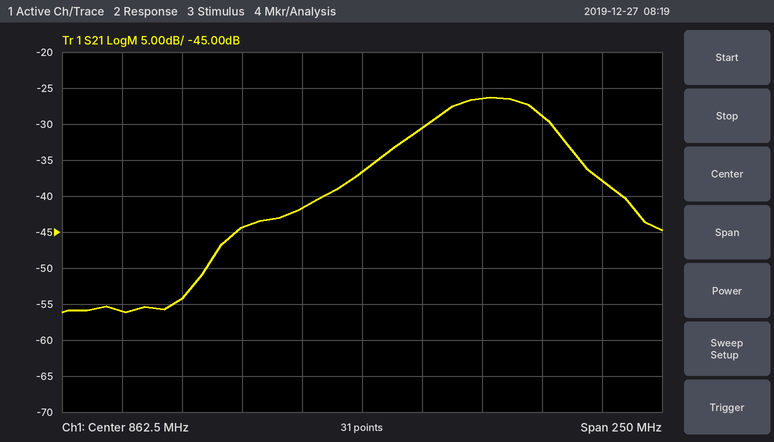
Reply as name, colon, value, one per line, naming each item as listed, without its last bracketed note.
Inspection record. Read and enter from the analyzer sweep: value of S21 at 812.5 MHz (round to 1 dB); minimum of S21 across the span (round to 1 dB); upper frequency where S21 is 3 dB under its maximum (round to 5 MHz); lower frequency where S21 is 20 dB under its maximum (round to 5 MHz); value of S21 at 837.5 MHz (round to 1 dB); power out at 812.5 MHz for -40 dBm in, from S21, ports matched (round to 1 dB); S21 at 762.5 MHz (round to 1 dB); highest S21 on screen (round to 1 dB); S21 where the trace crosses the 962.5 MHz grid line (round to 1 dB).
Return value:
value of S21 at 812.5 MHz: -44 dB
minimum of S21 across the span: -56 dB
upper frequency where S21 is 3 dB under its maximum: 940 MHz
lower frequency where S21 is 20 dB under its maximum: 805 MHz
value of S21 at 837.5 MHz: -42 dB
power out at 812.5 MHz for -40 dBm in, from S21, ports matched: -84 dBm
S21 at 762.5 MHz: -56 dB
highest S21 on screen: -26 dB
S21 where the trace crosses the 962.5 MHz grid line: -38 dB
